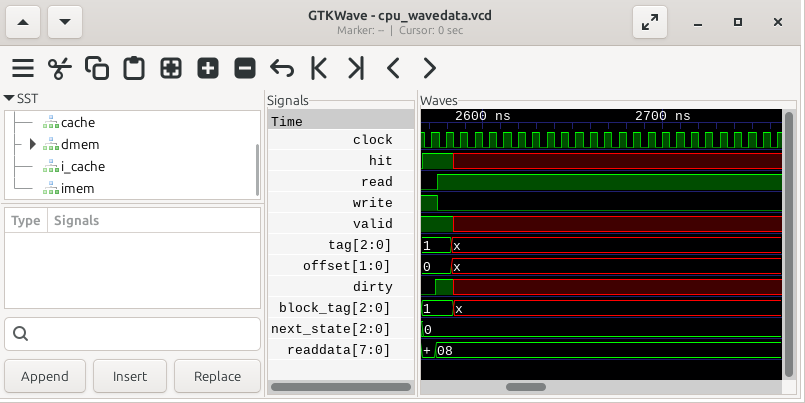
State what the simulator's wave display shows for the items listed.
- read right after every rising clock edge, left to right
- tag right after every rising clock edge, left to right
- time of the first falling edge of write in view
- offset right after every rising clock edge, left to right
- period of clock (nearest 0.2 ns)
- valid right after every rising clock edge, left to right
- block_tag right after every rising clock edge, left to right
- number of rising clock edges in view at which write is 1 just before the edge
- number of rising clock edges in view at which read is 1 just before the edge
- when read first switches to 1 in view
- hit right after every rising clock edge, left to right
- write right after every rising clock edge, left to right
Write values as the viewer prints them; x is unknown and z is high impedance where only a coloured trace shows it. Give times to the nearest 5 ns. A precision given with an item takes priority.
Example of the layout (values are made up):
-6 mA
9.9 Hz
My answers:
0 1 1 1 1 1 1 1 1 1 1 1 1 1 1 1 1 1 1 1 1 1 1 1 1
1, 1, x, x, x, x, x, x, x, x, x, x, x, x, x, x, x, x, x, x, x, x, x, x, x
2575 ns
0, 0, x, x, x, x, x, x, x, x, x, x, x, x, x, x, x, x, x, x, x, x, x, x, x
8 ns
1 1 x x x x x x x x x x x x x x x x x x x x x x x
1, 1, x, x, x, x, x, x, x, x, x, x, x, x, x, x, x, x, x, x, x, x, x, x, x
1
24
2575 ns
1 1 x x x x x x x x x x x x x x x x x x x x x x x
1 0 0 0 0 0 0 0 0 0 0 0 0 0 0 0 0 0 0 0 0 0 0 0 0
